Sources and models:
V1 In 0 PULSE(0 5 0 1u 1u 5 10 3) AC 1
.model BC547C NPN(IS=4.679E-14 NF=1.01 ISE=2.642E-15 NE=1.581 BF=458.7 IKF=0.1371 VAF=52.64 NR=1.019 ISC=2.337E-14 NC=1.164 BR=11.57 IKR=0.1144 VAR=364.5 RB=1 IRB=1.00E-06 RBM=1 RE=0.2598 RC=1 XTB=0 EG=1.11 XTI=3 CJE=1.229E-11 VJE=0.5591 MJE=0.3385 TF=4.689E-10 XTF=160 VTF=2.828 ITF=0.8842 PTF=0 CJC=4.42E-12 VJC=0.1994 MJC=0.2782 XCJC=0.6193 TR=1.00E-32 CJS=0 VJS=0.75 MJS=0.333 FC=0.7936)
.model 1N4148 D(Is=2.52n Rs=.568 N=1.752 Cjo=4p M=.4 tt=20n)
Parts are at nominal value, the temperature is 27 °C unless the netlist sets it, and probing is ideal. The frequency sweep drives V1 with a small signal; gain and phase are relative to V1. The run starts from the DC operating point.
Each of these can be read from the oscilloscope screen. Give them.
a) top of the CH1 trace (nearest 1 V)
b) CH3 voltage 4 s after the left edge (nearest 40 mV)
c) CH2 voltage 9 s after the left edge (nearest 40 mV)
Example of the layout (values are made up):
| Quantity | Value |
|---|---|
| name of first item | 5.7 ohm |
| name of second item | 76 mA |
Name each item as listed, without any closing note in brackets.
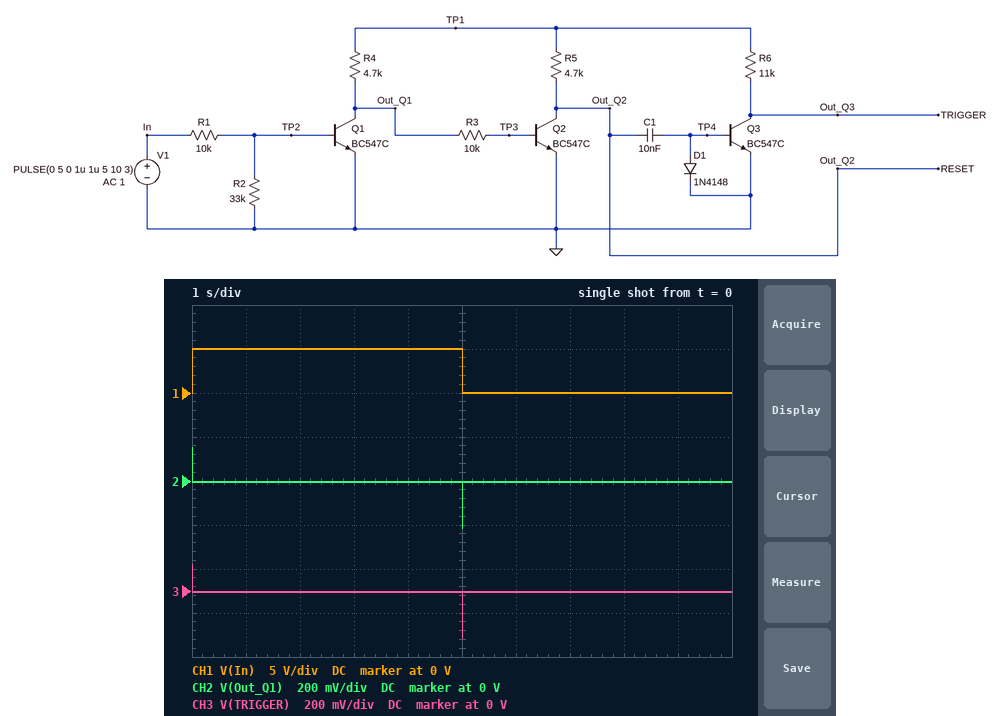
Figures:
| Quantity | Value |
|---|---|
| top of the CH1 trace | 5 V |
| CH3 voltage 4 s after the left edge | 0 V |
| CH2 voltage 9 s after the left edge | 0 V |
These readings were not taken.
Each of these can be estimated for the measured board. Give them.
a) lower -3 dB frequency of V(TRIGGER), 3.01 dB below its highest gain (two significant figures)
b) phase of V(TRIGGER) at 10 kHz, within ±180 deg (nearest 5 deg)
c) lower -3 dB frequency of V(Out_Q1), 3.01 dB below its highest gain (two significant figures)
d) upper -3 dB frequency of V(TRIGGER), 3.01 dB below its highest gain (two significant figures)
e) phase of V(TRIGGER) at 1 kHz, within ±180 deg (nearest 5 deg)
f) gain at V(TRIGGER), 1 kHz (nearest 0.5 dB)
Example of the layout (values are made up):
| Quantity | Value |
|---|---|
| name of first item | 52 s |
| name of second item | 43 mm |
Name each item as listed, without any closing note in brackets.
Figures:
| Quantity | Value |
|---|---|
| lower -3 dB frequency of V(TRIGGER), 3.01 dB below its highest gain | 270 Hz |
| phase of V(TRIGGER) at 10 kHz, within ±180 deg | 0 deg |
| lower -3 dB frequency of V(Out_Q1), 3.01 dB below its highest gain | 290 Hz |
| upper -3 dB frequency of V(TRIGGER), 3.01 dB below its highest gain | 2.4 MHz |
| phase of V(TRIGGER) at 1 kHz, within ±180 deg | 15 deg |
| gain at V(TRIGGER), 1 kHz | -20.0 dB |
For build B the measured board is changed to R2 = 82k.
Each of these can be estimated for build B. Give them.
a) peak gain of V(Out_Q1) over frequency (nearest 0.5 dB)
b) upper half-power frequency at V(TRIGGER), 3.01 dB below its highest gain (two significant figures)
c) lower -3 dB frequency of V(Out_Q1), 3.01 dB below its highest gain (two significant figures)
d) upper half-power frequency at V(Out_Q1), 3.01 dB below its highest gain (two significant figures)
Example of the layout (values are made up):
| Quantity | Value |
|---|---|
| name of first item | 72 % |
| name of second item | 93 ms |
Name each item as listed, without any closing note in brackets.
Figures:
| Quantity | Value |
|---|---|
| peak gain of V(Out_Q1) over frequency | -18.5 dB |
| upper half-power frequency at V(TRIGGER), 3.01 dB below its highest gain | 1.9 MHz |
| lower -3 dB frequency of V(Out_Q1), 3.01 dB below its highest gain | 270 Hz |
| upper half-power frequency at V(Out_Q1), 3.01 dB below its highest gain | 8.6 MHz |
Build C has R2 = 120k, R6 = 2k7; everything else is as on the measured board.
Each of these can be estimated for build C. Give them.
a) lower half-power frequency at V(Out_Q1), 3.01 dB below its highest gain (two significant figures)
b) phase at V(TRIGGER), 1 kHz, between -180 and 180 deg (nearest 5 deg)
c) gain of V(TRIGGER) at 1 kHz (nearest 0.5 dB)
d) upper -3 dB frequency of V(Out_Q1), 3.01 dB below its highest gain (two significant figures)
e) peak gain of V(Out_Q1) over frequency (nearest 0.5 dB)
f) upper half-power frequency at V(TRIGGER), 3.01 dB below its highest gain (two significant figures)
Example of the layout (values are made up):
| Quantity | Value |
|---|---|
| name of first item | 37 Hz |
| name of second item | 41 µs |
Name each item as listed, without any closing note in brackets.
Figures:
| Quantity | Value |
|---|---|
| lower half-power frequency at V(Out_Q1), 3.01 dB below its highest gain | 270 Hz |
| phase at V(TRIGGER), 1 kHz, between -180 and 180 deg | 15 deg |
| gain of V(TRIGGER) at 1 kHz | -18.5 dB |
| upper -3 dB frequency of V(Out_Q1), 3.01 dB below its highest gain | 6.7 MHz |
| peak gain of V(Out_Q1) over frequency | -18.0 dB |
| upper half-power frequency at V(TRIGGER), 3.01 dB below its highest gain | 1.6 MHz |
